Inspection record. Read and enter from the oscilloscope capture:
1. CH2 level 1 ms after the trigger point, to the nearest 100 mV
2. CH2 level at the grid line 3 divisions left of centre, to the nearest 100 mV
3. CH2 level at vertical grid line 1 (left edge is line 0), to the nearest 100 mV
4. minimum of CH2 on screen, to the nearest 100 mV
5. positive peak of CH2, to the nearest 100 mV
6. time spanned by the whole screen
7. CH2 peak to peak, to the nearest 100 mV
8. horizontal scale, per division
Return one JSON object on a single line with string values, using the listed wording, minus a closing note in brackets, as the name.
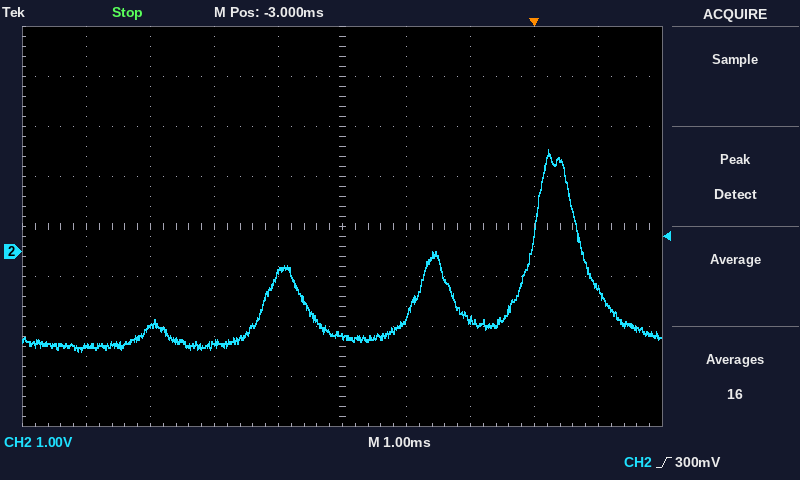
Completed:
{"CH2 level 1 ms after the trigger point, to the nearest 100 mV": "-700 mV", "CH2 level at the grid line 3 divisions left of centre, to the nearest 100 mV": "-1.5 V", "CH2 level at vertical grid line 1 (left edge is line 0), to the nearest 100 mV": "-1.9 V", "minimum of CH2 on screen, to the nearest 100 mV": "-2.0 V", "positive peak of CH2, to the nearest 100 mV": "2.0 V", "time spanned by the whole screen": "10 ms", "CH2 peak to peak, to the nearest 100 mV": "4.0 V", "horizontal scale, per division": "1 ms"}
